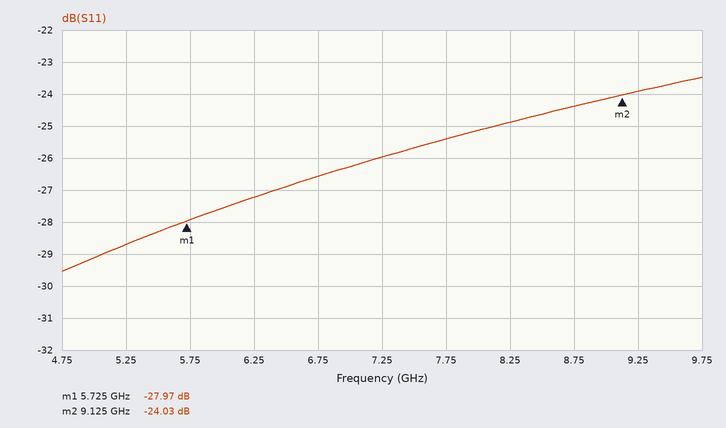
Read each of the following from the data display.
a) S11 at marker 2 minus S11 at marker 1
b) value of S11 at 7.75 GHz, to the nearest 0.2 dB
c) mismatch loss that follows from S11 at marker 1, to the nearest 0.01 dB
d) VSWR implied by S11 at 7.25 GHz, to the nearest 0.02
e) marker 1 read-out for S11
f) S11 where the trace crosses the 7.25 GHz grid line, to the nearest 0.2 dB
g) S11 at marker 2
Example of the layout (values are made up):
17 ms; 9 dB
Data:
3.94 dB; -25.4 dB; 0.01 dB; 1.10; -27.97 dB; -26.0 dB; -24.03 dB
